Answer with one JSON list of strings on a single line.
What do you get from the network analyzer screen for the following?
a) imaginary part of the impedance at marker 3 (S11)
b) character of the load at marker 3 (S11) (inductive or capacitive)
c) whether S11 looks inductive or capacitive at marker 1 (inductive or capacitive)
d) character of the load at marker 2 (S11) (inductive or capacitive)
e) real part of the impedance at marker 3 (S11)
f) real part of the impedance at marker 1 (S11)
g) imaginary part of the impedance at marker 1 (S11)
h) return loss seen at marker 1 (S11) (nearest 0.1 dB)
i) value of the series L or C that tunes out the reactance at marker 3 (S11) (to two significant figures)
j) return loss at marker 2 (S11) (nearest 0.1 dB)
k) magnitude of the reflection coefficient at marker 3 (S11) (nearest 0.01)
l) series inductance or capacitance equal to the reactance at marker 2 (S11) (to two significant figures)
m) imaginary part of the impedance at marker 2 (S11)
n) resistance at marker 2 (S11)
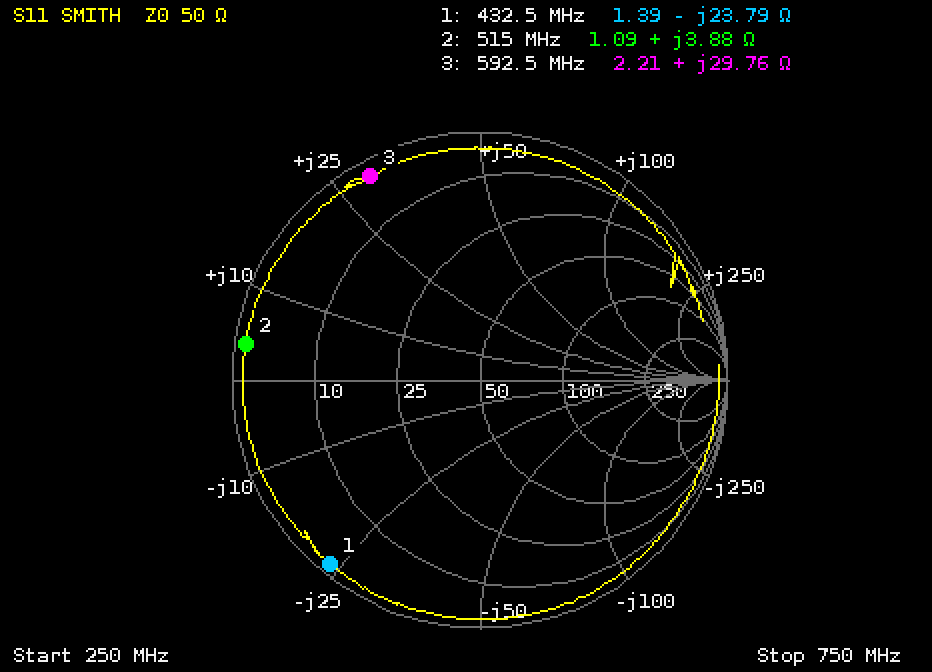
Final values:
["+29.76 Ω", "inductive", "capacitive", "inductive", "2.21 Ω", "1.39 Ω", "-23.79 Ω", "0.4 dB", "9.0 pF", "0.4 dB", "0.94", "1.2 nH", "+3.88 Ω", "1.09 Ω"]
